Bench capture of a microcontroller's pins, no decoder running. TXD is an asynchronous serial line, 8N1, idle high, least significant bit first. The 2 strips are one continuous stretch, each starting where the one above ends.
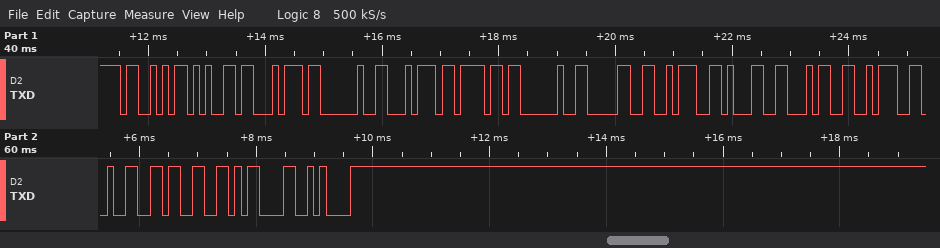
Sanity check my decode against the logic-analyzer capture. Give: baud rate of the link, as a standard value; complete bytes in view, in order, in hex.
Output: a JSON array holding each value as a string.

["9600 baud", "53 65 74 20 74 6F 20 30 3A 31 34 3A 32 33 0D 0A"]
